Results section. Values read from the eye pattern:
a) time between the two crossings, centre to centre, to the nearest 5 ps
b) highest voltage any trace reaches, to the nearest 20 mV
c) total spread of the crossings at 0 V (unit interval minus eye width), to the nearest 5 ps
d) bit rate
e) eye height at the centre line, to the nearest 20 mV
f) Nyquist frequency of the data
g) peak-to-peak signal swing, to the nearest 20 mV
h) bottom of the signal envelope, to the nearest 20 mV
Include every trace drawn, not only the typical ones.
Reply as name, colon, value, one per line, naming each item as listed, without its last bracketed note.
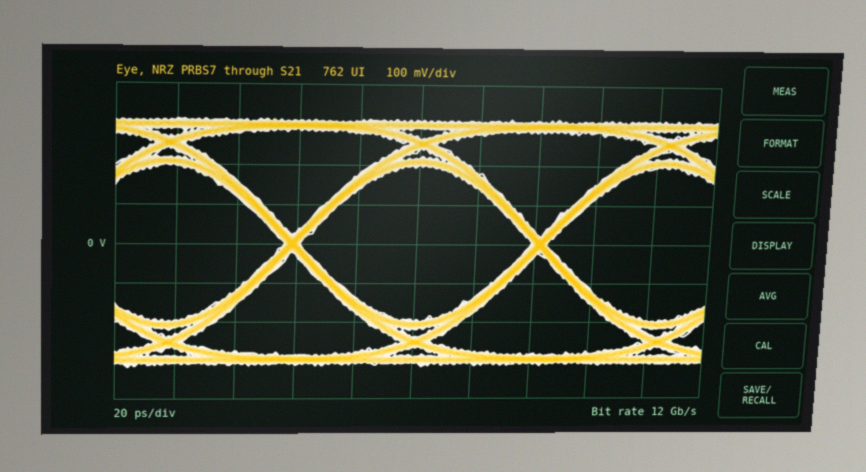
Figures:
time between the two crossings, centre to centre, to the nearest 5 ps: 85 ps
highest voltage any trace reaches, to the nearest 20 mV: 320 mV
total spread of the crossings at 0 V (unit interval minus eye width), to the nearest 5 ps: 5 ps
bit rate: 12 Gb/s
eye height at the centre line, to the nearest 20 mV: 400 mV
Nyquist frequency of the data: 6 GHz
peak-to-peak signal swing, to the nearest 20 mV: 640 mV
bottom of the signal envelope, to the nearest 20 mV: -320 mV
